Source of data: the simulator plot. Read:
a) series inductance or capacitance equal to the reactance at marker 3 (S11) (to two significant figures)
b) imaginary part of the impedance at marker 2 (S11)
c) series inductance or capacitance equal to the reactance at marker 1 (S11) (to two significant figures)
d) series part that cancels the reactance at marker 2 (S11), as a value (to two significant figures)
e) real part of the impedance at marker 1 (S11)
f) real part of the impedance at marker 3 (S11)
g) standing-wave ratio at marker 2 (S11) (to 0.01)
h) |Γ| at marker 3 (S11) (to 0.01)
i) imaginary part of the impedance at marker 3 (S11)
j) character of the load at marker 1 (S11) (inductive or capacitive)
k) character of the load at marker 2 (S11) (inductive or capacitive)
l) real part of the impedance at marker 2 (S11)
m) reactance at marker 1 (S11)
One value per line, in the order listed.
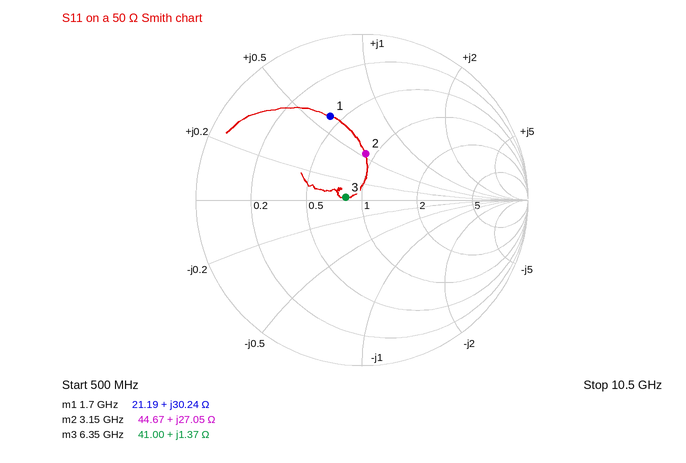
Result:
34 pH
+27.05 Ω
2.8 nH
1.9 pF
21.19 Ω
41.00 Ω
1.78
0.10
+1.37 Ω
inductive
inductive
44.67 Ω
+30.24 Ω
